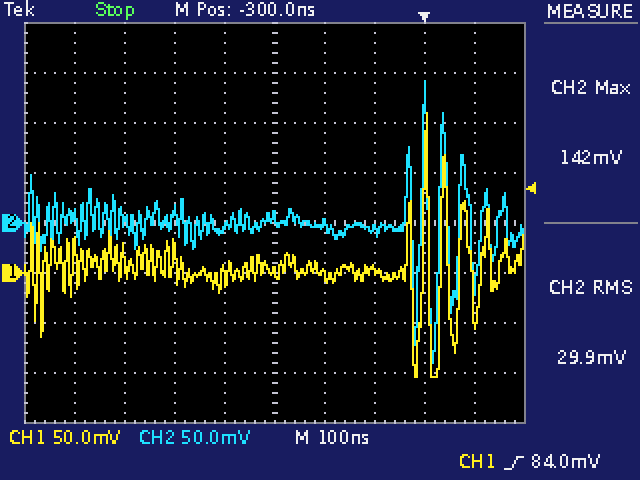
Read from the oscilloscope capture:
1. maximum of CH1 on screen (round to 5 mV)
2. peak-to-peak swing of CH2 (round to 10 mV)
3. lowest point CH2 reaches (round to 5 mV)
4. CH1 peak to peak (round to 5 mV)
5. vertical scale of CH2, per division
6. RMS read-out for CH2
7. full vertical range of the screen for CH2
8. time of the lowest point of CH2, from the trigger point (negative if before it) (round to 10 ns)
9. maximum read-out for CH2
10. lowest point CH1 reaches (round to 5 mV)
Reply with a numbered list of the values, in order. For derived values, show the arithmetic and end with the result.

1. 160 mV
2. 280 mV
3. -140 mV
4. 160 mV − (-105 mV) = 265 mV
5. 50 mV
6. 29.9 mV
7. 400 mV
8. +20 ns
9. 142 mV
10. -105 mV
